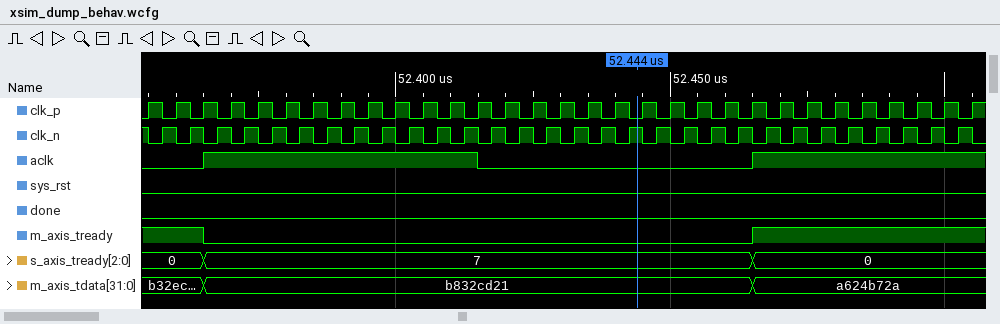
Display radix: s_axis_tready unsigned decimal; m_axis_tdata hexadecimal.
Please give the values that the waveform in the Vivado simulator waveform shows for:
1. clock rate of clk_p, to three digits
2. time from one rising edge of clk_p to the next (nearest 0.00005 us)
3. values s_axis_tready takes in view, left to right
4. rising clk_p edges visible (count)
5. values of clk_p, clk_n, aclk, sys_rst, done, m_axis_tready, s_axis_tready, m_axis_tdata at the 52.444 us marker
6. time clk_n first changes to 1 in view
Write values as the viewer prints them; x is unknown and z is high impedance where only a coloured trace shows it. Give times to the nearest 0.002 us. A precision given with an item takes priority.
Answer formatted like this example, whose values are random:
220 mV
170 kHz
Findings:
200 MHz
0.005 us
0, 7, 0
31
clk_p=0, clk_n=1, aclk=0, sys_rst=0, done=0, m_axis_tready=0, s_axis_tready=7, m_axis_tdata=b832cd21
52.358 us
